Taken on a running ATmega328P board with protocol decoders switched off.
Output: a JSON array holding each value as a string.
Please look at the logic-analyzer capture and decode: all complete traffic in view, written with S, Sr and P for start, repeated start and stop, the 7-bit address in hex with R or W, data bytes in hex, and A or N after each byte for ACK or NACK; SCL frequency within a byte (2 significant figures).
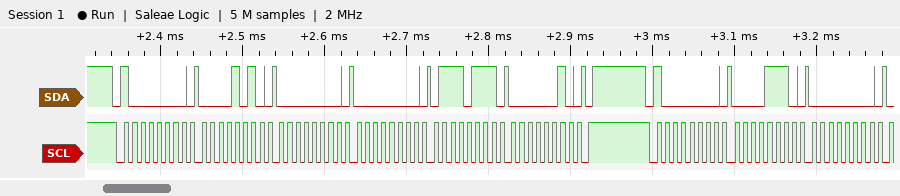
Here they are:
["S 40W A 0A A 00 A 00 A 77 A 02 A P S 40W A 0E A 00 A", "100 kHz"]
